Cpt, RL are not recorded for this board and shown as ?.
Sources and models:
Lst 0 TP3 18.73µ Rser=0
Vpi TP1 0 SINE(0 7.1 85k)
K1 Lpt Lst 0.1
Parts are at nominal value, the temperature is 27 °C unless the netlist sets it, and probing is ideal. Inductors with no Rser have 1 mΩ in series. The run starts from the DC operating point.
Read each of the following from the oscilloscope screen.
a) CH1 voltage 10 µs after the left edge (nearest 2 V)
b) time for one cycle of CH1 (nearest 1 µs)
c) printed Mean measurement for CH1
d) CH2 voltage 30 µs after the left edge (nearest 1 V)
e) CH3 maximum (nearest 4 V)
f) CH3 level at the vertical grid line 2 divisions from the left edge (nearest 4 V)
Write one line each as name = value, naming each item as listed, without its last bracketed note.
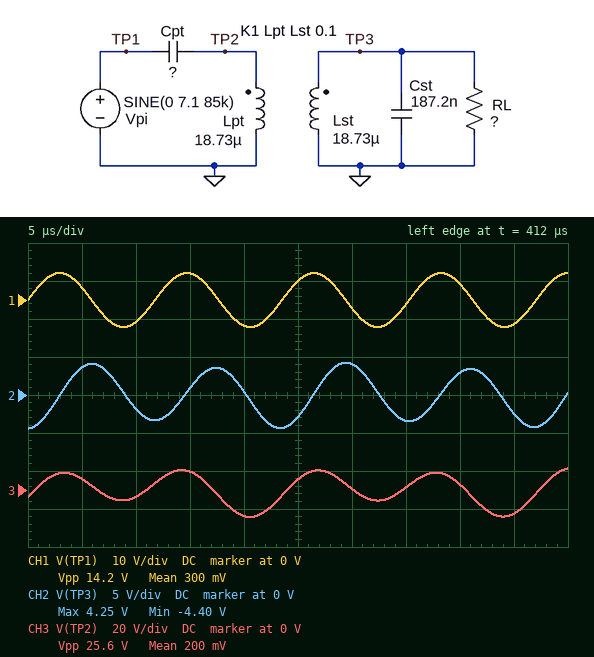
CH1 voltage 10 µs after the left edge = -6 V
time for one cycle of CH1 = 12 µs
printed Mean measurement for CH1 = 300 mV
CH2 voltage 30 µs after the left edge = 4 V
CH3 maximum = 12 V
CH3 level at the vertical grid line 2 divisions from the left edge = -4 V
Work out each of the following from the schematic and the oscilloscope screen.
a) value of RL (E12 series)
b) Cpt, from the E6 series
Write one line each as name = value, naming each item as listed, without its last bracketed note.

value of RL = 39 Ω
Cpt, from the E6 series = 680 nF
